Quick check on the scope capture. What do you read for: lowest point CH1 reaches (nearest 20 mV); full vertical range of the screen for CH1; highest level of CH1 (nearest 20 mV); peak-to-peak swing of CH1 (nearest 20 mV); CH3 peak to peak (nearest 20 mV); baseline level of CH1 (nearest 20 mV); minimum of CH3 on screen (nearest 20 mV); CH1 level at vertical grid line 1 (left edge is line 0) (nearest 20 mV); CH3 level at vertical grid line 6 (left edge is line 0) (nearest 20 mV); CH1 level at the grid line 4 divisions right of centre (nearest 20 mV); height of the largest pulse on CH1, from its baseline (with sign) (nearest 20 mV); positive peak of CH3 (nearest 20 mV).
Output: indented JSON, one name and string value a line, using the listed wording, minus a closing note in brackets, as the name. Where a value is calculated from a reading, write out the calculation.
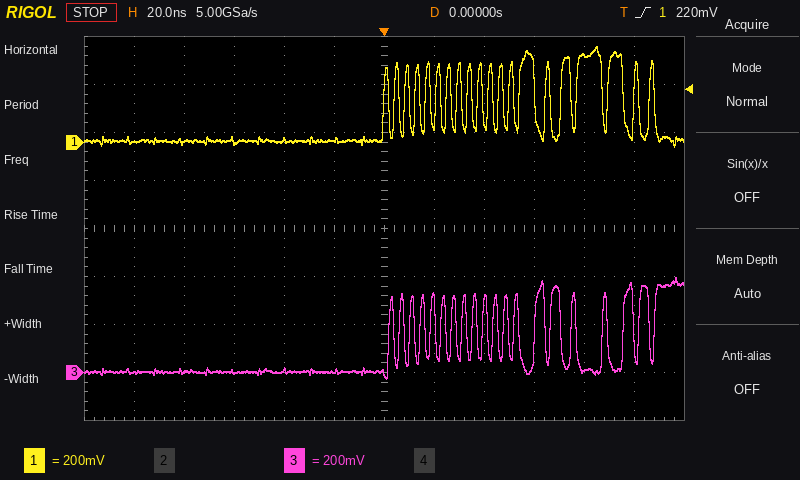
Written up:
{
  "lowest point CH1 reaches": "-20 mV",
  "full vertical range of the screen for CH1": "1.6 V",
  "highest level of CH1": "400 mV",
  "peak-to-peak swing of CH1": "400 mV − (-20 mV) = 420 mV",
  "CH3 peak to peak": "400 mV − (-20 mV) = 420 mV",
  "baseline level of CH1": "0 mV",
  "minimum of CH3 on screen": "-20 mV",
  "CH1 level at vertical grid line 1 (left edge is line 0)": "0 mV",
  "CH3 level at vertical grid line 6 (left edge is line 0)": "0 mV",
  "CH1 level at the grid line 4 divisions right of centre": "360 mV",
  "height of the largest pulse on CH1, from its baseline (with sign)": "400 mV − (0 mV) = +400 mV",
  "positive peak of CH3": "400 mV"
}
